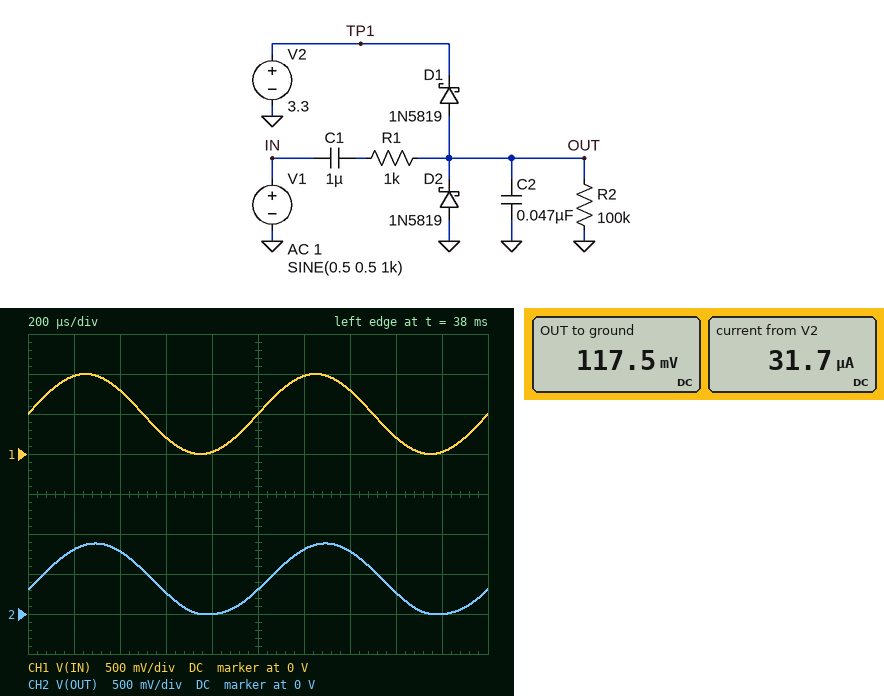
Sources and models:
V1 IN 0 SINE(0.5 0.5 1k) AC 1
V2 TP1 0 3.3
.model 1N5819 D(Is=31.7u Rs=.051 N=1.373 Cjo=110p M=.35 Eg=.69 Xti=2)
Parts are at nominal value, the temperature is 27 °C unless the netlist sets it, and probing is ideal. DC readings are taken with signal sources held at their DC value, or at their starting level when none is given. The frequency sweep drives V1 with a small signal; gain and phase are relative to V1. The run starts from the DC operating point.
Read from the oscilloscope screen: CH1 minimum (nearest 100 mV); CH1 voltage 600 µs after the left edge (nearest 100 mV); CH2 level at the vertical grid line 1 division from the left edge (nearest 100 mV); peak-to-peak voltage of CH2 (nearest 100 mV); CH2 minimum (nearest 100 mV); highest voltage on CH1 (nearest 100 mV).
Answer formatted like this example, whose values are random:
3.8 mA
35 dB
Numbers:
0 V
200 mV
800 mV
900 mV
0 V
1.0 V
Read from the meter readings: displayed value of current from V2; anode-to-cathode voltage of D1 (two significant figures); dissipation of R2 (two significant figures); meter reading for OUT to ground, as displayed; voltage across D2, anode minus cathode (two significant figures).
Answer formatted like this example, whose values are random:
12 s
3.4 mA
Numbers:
31.7 µA
-3.2 V
140 nW
117.5 mV
-120 mV
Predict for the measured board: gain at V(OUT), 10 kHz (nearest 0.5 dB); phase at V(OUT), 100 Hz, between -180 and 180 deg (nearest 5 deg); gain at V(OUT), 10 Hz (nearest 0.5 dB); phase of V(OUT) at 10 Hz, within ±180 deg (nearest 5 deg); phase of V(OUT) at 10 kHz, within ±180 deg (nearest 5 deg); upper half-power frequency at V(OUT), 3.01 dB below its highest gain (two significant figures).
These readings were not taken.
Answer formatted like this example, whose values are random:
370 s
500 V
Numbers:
-10.0 dB
0 deg
-2.0 dB
30 deg
-70 deg
3.7 kHz
